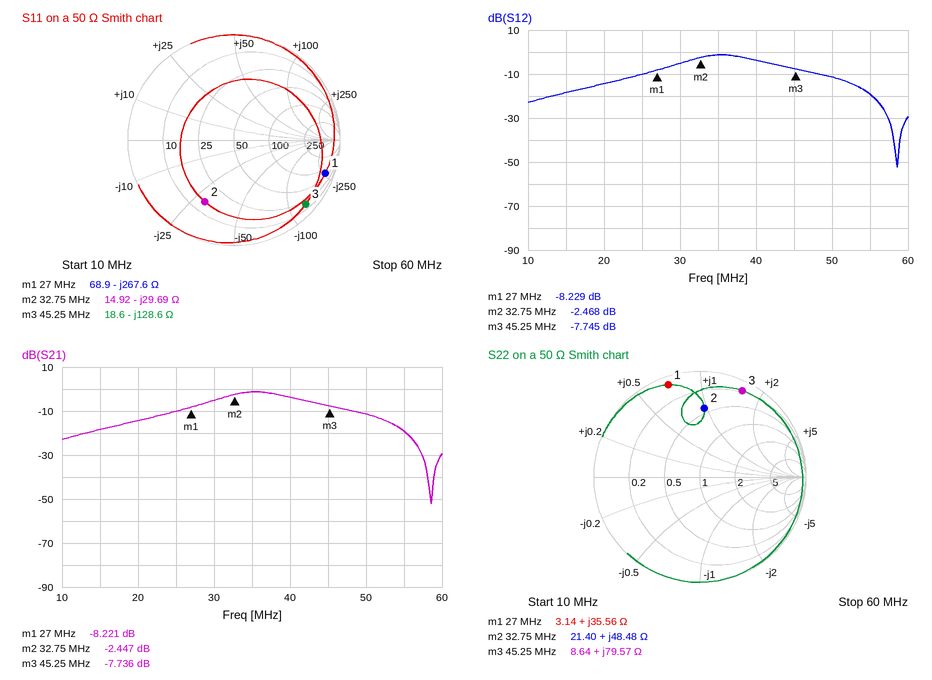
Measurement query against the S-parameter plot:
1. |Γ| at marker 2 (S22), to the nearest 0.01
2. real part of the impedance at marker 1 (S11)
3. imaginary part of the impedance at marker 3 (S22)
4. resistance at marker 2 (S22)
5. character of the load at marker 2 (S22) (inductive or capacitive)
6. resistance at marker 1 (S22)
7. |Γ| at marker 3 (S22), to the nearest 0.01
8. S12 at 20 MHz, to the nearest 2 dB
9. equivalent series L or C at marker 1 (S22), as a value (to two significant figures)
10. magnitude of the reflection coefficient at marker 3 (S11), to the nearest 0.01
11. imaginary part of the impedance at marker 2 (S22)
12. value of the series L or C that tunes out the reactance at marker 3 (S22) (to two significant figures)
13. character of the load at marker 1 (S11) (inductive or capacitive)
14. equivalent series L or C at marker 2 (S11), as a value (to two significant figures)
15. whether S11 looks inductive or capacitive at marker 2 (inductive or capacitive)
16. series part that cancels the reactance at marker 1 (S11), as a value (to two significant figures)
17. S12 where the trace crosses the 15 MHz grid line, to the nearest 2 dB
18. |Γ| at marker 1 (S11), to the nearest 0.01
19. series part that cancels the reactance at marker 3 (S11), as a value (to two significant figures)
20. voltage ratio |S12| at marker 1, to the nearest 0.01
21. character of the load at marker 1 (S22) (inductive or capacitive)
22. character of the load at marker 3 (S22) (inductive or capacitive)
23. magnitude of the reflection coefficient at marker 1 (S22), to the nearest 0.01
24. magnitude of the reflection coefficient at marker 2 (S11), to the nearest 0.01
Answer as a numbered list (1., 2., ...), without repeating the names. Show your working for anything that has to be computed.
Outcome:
1. 0.65
2. 68.9 Ω
3. +79.57 Ω
4. 21.40 Ω
5. inductive
6. 3.14 Ω
7. 0.91
8. -14 dB
9. L = 35.56 Ω/(2π × 27 MHz) ≈ 210 nH
10. 0.91
11. +48.48 Ω
12. C = 1/(2π × 45.25 MHz × 79.57 Ω) ≈ 44 pF
13. capacitive
14. C = 1/(2π × 32.75 MHz × 29.69 Ω) ≈ 164 pF, so 160 pF to two significant figures
15. capacitive
16. L = 267.6 Ω/(2π × 27 MHz) ≈ 1.6 µH
17. -18 dB
18. 0.92
19. L = 128.6 Ω/(2π × 45.25 MHz) ≈ 452 nH, so 450 nH to two significant figures
20. 10^(-8.229/20) ≈ 0.39
21. inductive
22. inductive
23. 0.92
24. 0.64
